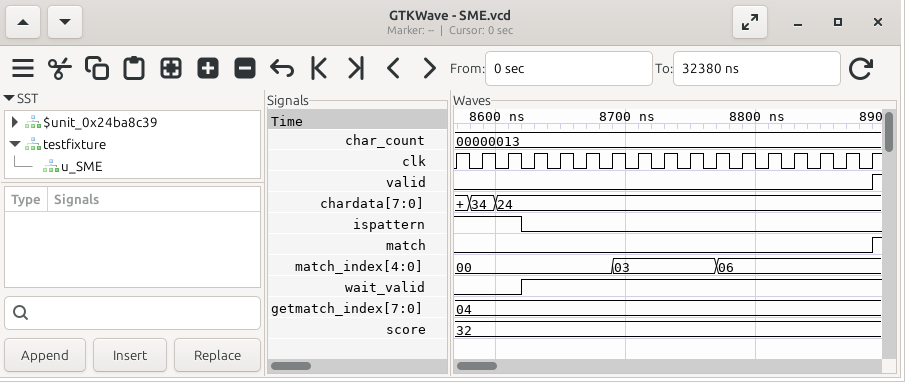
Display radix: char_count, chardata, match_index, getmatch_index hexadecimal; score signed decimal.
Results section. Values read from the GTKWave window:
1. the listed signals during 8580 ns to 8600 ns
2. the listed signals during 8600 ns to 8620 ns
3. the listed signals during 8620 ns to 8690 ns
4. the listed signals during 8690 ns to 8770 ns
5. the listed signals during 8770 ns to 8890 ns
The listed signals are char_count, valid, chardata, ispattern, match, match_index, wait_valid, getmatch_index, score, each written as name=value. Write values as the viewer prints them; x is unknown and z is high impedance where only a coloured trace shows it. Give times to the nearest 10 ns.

char_count=00000013, valid=0, chardata=34, ispattern=1, match=0, match_index=00, wait_valid=0, getmatch_index=04, score=32
char_count=00000013, valid=0, chardata=24, ispattern=1, match=0, match_index=00, wait_valid=0, getmatch_index=04, score=32
char_count=00000013, valid=0, chardata=24, ispattern=0, match=0, match_index=00, wait_valid=1, getmatch_index=04, score=32
char_count=00000013, valid=0, chardata=24, ispattern=0, match=0, match_index=03, wait_valid=1, getmatch_index=04, score=32
char_count=00000013, valid=0, chardata=24, ispattern=0, match=0, match_index=06, wait_valid=1, getmatch_index=04, score=32
